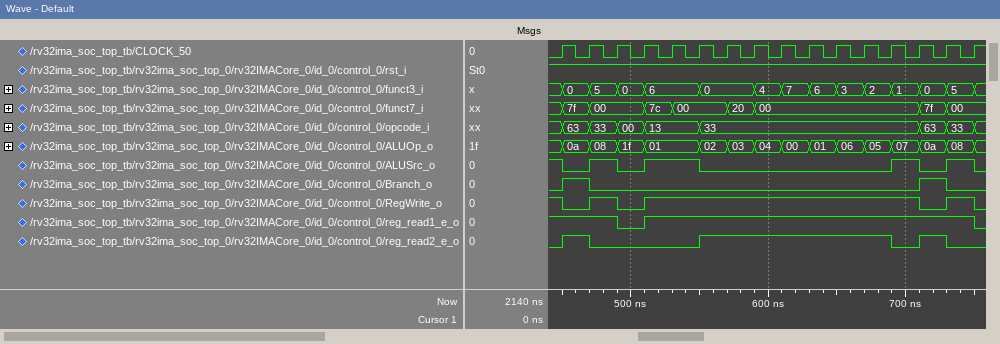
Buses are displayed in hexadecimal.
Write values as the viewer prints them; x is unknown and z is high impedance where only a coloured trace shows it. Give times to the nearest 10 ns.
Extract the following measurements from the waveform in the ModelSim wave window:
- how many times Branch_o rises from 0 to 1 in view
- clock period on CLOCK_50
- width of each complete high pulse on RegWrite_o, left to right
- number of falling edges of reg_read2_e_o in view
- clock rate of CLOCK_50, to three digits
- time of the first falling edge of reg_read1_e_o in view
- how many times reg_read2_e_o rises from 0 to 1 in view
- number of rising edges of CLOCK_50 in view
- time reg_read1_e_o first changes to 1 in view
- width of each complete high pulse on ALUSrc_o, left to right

2
20 ns
20 ns, 200 ns, 20 ns
3
50.0 MHz
490 ns
3
16
510 ns
20 ns, 40 ns, 20 ns, 20 ns
